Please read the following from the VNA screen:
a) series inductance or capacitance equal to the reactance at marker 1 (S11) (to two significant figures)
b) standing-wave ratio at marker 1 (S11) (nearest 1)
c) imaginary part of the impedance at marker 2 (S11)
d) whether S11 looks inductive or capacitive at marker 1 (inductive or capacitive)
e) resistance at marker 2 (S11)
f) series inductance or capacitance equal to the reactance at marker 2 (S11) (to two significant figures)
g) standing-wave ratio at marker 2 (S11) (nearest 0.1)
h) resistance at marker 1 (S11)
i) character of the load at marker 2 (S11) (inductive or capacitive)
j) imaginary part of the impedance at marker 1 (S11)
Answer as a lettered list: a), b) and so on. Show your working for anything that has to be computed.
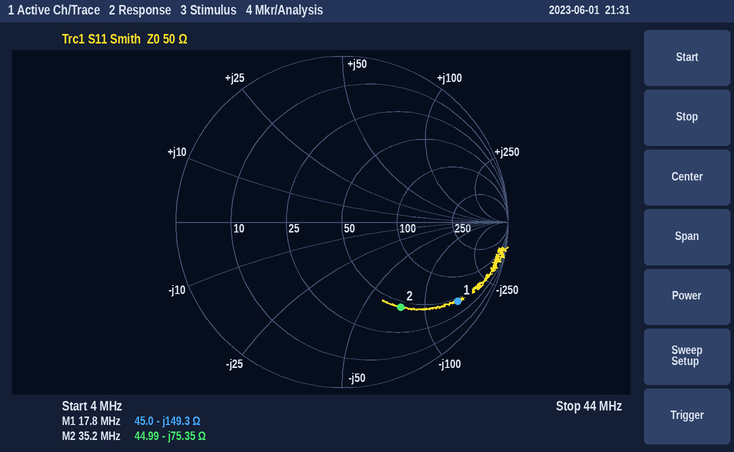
a) C = 1/(2π × 17.8 MHz × 149.3 Ω) ≈ 60 pF
b) 12
c) -75.35 Ω
d) capacitive
e) 44.99 Ω
f) C = 1/(2π × 35.2 MHz × 75.35 Ω) ≈ 60 pF
g) 4.3
h) 45.0 Ω
i) capacitive
j) -149.3 Ω
